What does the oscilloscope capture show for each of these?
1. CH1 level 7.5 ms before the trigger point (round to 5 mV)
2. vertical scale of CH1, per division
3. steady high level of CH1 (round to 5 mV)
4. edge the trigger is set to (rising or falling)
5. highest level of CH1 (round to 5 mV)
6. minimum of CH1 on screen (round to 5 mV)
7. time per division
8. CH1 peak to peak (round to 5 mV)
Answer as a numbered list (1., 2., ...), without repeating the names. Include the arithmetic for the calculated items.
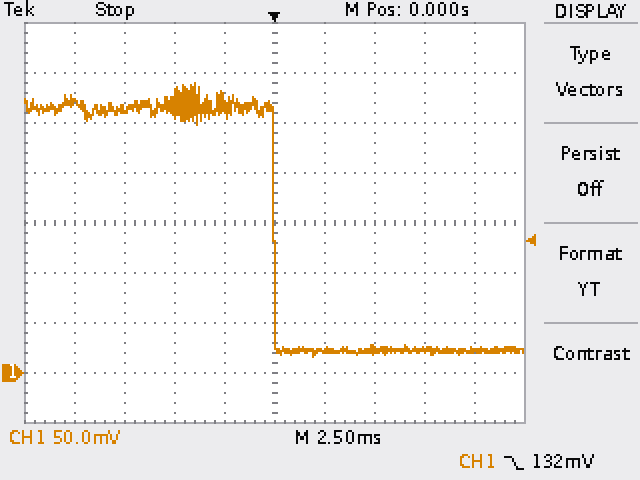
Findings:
1. 265 mV
2. 50 mV
3. 265 mV
4. falling
5. 290 mV
6. 15 mV
7. 2.5 ms
8. 290 mV − (15 mV) = 275 mV
